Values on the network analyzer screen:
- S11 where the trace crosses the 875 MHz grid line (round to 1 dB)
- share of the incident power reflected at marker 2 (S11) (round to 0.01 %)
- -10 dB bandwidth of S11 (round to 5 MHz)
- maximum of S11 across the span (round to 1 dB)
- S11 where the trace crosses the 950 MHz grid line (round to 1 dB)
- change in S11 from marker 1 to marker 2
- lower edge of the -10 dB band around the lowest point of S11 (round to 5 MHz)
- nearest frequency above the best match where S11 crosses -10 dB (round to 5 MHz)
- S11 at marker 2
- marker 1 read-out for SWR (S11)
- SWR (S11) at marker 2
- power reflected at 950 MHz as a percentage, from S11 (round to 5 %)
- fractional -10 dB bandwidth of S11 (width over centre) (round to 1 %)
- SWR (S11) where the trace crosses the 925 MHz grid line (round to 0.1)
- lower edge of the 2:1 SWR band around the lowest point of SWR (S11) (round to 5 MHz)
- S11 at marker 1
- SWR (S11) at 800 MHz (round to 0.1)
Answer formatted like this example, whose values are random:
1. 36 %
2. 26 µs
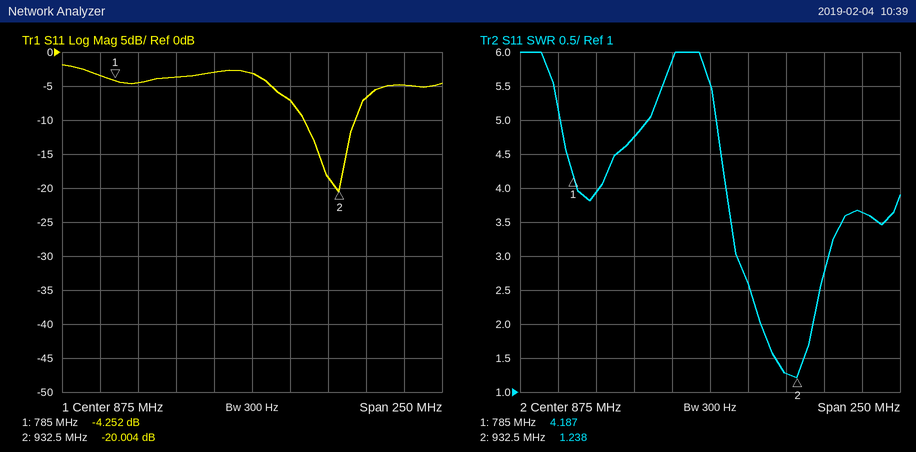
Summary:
1. -3 dB
2. 1.00 %
3. 35 MHz
4. -2 dB
5. -7 dB
6. -15.752 dB
7. 910 MHz
8. 945 MHz
9. -20.004 dB
10. 4.187
11. 1.238
12. 20 %
13. 4 %
14. 1.3
15. 910 MHz
16. -4.252 dB
17. 3.9
